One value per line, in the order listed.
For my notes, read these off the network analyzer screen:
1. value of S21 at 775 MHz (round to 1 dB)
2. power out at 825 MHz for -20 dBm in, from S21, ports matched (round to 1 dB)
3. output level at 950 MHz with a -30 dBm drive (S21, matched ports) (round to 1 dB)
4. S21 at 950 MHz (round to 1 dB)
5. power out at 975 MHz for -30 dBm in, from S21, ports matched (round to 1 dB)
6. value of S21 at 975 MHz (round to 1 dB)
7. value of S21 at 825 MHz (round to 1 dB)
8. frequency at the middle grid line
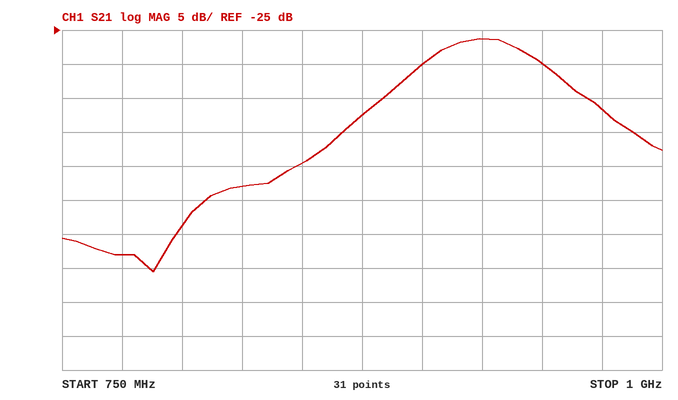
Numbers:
-58 dB
-68 dBm
-60 dBm
-30 dB
-67 dBm
-37 dB
-48 dB
875 MHz
